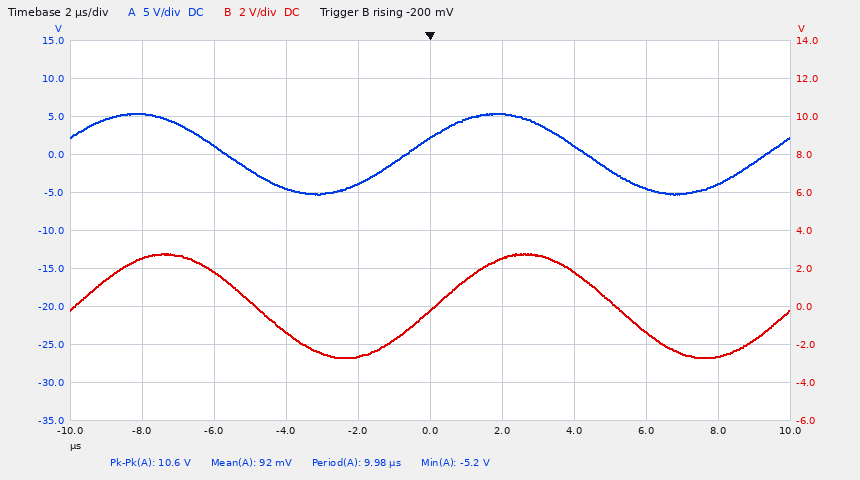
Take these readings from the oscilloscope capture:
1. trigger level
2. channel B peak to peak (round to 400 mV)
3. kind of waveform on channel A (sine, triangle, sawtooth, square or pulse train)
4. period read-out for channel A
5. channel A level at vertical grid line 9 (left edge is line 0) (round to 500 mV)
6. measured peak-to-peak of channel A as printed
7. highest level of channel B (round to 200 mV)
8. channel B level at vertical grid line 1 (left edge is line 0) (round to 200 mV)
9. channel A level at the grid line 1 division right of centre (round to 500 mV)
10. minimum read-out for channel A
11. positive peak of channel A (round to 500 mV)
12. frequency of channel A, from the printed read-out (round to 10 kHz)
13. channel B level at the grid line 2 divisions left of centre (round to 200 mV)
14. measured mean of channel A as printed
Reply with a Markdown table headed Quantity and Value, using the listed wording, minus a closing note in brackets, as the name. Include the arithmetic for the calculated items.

| Quantity | Value |
|---|---|
| trigger level | -200 mV |
| channel B peak to peak | 5.6 V |
| kind of waveform on channel A | sine |
| period read-out for channel A | 9.98 µs |
| channel A level at vertical grid line 9 (left edge is line 0) | -4.0 V |
| measured peak-to-peak of channel A as printed | 10.6 V |
| highest level of channel B | 2.8 V |
| channel B level at vertical grid line 1 (left edge is line 0) | 2.6 V |
| channel A level at the grid line 1 division right of centre | 5.5 V |
| minimum read-out for channel A | -5.2 V |
| positive peak of channel A | 5.5 V |
| frequency of channel A, from the printed read-out | 1 / 9.98 µs ≈ 100 kHz |
| channel B level at the grid line 2 divisions left of centre | -1.4 V |
| measured mean of channel A as printed | 92 mV |
